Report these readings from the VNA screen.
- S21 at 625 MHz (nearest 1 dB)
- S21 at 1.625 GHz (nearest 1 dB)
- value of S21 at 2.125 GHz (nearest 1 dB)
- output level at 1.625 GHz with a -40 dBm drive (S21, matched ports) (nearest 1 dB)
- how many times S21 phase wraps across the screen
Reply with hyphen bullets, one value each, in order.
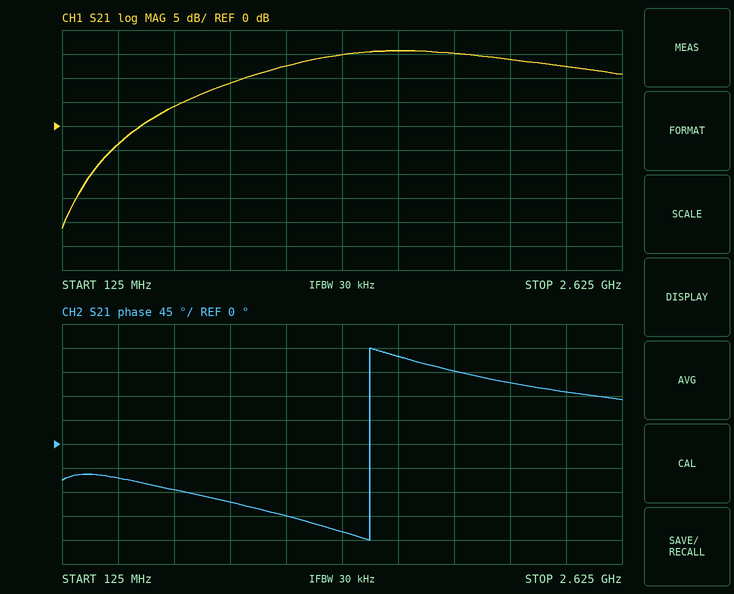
- 4 dB
- 16 dB
- 14 dB
- -24 dBm
- 1
